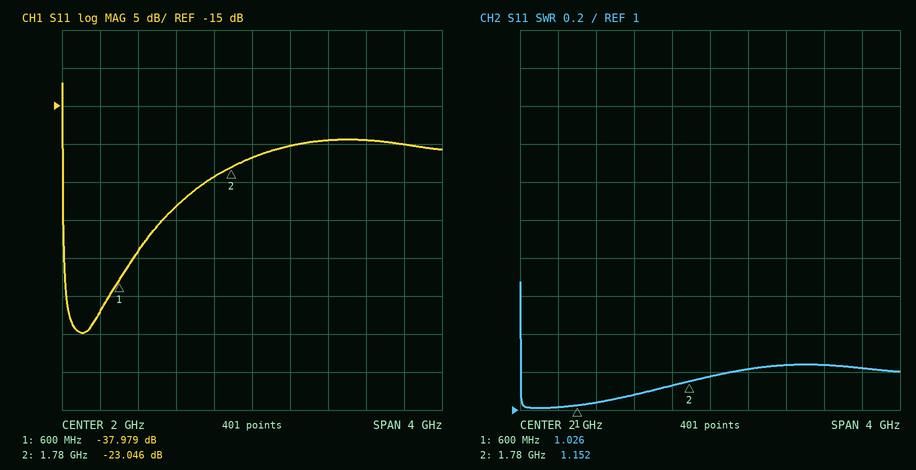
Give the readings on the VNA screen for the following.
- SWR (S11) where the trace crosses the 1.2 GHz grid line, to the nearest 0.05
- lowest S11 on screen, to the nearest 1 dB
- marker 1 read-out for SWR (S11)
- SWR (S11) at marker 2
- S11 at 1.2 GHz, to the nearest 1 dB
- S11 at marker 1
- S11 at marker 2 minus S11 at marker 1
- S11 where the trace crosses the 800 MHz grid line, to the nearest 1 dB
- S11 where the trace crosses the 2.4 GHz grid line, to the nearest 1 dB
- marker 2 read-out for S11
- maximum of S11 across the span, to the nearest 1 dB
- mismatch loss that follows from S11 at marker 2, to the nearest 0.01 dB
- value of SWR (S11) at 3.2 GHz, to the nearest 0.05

1.10
-45 dB
1.026
1.152
-28 dB
-37.979 dB
14.933 dB
-34 dB
-20 dB
-23.046 dB
-12 dB
0.02 dB
1.25
